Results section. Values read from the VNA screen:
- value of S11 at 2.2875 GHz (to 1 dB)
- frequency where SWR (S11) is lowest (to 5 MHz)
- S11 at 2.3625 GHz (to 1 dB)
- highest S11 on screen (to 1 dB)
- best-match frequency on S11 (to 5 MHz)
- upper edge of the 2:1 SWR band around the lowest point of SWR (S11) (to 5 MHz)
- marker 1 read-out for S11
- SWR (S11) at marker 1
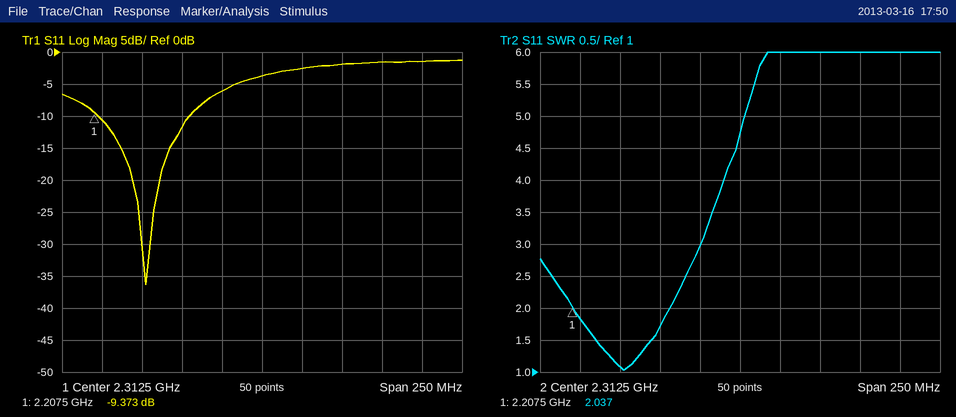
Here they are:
-6 dB
2.240 GHz
-2 dB
-1 dB
2.240 GHz
2.270 GHz
-9.373 dB
2.037
